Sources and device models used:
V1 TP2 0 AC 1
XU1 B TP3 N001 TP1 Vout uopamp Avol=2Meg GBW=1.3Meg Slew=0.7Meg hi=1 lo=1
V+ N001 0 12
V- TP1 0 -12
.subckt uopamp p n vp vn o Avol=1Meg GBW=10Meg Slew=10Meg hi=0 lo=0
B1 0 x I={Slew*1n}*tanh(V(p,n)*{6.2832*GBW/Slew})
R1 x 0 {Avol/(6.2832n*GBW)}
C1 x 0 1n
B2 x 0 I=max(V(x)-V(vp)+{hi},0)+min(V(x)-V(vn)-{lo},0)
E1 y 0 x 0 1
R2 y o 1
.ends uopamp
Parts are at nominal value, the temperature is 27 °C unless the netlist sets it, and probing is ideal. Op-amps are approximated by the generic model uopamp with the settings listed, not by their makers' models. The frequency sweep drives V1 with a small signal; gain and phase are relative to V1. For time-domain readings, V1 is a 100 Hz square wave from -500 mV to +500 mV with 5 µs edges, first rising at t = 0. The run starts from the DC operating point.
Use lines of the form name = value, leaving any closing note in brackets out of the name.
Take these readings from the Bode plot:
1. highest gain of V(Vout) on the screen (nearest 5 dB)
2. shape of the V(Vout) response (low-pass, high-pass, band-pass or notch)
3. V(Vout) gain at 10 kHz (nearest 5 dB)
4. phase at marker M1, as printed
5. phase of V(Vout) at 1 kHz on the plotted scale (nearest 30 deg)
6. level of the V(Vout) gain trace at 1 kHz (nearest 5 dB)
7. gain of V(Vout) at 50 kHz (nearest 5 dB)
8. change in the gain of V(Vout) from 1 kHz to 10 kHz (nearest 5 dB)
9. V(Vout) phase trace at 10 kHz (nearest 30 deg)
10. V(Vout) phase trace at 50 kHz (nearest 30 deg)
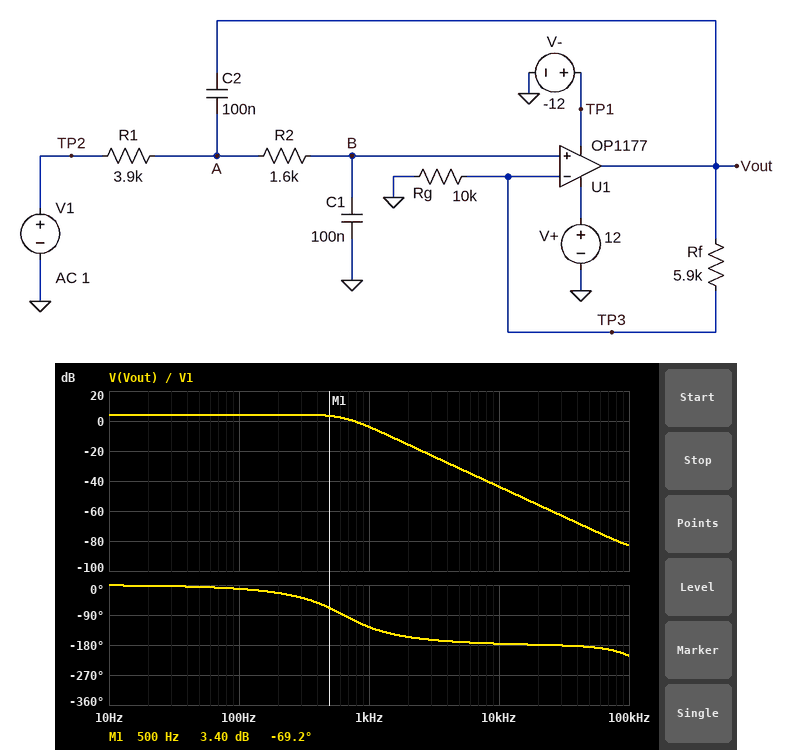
highest gain of V(Vout) on the screen = 5 dB
shape of the V(Vout) response = low-pass
V(Vout) gain at 10 kHz = -45 dB
phase at marker M1, as printed = -69.2 deg
phase of V(Vout) at 1 kHz on the plotted scale = -120 deg
level of the V(Vout) gain trace at 1 kHz = -5 dB
gain of V(Vout) at 50 kHz = -70 dB
change in the gain of V(Vout) from 1 kHz to 10 kHz = -40 dB
V(Vout) phase trace at 10 kHz = -180 deg
V(Vout) phase trace at 50 kHz = -180 deg
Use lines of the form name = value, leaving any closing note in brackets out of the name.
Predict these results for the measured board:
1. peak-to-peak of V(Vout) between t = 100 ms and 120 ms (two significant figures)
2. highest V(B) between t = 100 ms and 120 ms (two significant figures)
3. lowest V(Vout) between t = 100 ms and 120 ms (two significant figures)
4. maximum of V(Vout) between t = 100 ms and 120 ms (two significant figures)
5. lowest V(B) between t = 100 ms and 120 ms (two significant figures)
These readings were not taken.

peak-to-peak of V(Vout) between t = 100 ms and 120 ms = 1.8 V
highest V(B) between t = 100 ms and 120 ms = 570 mV
lowest V(Vout) between t = 100 ms and 120 ms = -910 mV
maximum of V(Vout) between t = 100 ms and 120 ms = 910 mV
lowest V(B) between t = 100 ms and 120 ms = -570 mV
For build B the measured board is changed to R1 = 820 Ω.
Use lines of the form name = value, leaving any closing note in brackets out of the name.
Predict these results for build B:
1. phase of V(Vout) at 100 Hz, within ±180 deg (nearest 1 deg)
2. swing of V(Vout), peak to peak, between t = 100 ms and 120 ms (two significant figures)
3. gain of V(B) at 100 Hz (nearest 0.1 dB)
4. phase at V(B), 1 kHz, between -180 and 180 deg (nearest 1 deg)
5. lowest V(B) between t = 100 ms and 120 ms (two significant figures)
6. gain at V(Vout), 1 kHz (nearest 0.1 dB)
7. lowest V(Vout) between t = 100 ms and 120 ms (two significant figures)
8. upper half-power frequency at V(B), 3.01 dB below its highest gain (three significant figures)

phase of V(Vout) at 100 Hz, within ±180 deg = -7 deg
swing of V(Vout), peak to peak, between t = 100 ms and 120 ms = 1.6 V
gain of V(B) at 100 Hz = 0 dB
phase at V(B), 1 kHz, between -180 and 180 deg = -68 deg
lowest V(B) between t = 100 ms and 120 ms = -510 mV
gain at V(Vout), 1 kHz = 1.7 dB
lowest V(Vout) between t = 100 ms and 120 ms = -810 mV
upper half-power frequency at V(B), 3.01 dB below its highest gain = 1.13 kHz
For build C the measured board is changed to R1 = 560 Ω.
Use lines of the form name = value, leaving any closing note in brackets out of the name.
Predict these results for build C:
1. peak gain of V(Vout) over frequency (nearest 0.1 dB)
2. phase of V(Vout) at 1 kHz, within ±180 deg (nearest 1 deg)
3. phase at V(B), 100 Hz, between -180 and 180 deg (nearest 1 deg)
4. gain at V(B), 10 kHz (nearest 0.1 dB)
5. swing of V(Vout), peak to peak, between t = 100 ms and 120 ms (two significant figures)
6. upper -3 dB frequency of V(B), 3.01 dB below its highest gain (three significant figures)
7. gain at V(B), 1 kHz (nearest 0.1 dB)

peak gain of V(Vout) over frequency = 4.0 dB
phase of V(Vout) at 1 kHz, within ±180 deg = -61 deg
phase at V(B), 100 Hz, between -180 and 180 deg = -7 deg
gain at V(B), 10 kHz = -31.2 dB
swing of V(Vout), peak to peak, between t = 100 ms and 120 ms = 1.6 V
upper -3 dB frequency of V(B), 3.01 dB below its highest gain = 1.14 kHz
gain at V(B), 1 kHz = -2.4 dB
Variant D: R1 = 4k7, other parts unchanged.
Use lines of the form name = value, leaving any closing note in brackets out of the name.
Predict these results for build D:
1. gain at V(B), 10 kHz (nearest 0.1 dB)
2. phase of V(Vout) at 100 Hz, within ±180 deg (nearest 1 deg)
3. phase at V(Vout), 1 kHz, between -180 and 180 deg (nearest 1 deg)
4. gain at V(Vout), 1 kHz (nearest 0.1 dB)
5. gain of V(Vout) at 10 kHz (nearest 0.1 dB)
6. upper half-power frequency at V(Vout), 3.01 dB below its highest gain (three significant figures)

gain at V(B), 10 kHz = -49.5 dB
phase of V(Vout) at 100 Hz, within ±180 deg = -13 deg
phase at V(Vout), 1 kHz, between -180 and 180 deg = -132 deg
gain at V(Vout), 1 kHz = -5.4 dB
gain of V(Vout) at 10 kHz = -45.4 dB
upper half-power frequency at V(Vout), 3.01 dB below its highest gain = 624 Hz
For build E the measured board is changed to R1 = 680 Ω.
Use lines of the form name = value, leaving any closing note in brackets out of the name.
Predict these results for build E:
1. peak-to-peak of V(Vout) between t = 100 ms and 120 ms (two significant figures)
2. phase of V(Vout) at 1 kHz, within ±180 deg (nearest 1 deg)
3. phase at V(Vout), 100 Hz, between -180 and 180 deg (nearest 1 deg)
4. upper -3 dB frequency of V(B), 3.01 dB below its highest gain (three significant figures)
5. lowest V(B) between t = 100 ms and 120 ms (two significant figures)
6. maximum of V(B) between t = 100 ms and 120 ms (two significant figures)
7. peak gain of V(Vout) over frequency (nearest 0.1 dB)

peak-to-peak of V(Vout) between t = 100 ms and 120 ms = 1.6 V
phase of V(Vout) at 1 kHz, within ±180 deg = -64 deg
phase at V(Vout), 100 Hz, between -180 and 180 deg = -7 deg
upper -3 dB frequency of V(B), 3.01 dB below its highest gain = 1.14 kHz
lowest V(B) between t = 100 ms and 120 ms = -500 mV
maximum of V(B) between t = 100 ms and 120 ms = 500 mV
peak gain of V(Vout) over frequency = 4.0 dB
